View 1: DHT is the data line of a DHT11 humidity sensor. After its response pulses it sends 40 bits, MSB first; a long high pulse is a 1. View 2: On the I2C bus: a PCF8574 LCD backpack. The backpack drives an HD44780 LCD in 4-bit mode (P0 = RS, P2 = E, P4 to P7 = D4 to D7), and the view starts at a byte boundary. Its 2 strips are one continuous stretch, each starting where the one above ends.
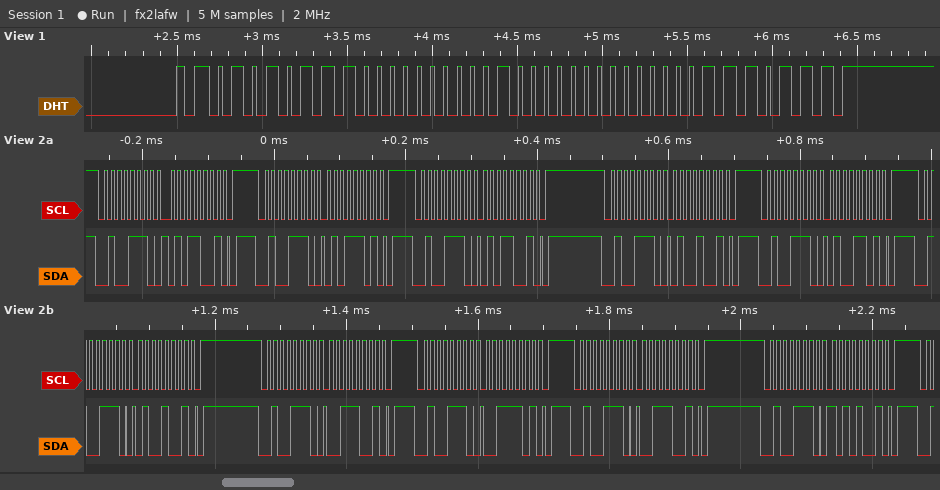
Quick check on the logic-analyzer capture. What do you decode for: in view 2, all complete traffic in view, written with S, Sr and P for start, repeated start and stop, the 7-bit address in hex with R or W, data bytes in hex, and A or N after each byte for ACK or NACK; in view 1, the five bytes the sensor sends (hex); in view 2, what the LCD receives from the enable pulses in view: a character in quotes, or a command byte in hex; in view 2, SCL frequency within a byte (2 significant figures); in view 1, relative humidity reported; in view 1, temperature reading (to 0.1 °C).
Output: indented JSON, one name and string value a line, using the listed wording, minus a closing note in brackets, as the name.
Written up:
{
  "in view 2, all complete traffic in view, written with S, Sr and P for start, repeated start and stop, the 7-bit address in hex with R or W, data bytes in hex, and A or N after each byte for ACK or NACK": "S 27W A 59 A P S 27W A 5D A P S 27W A 59 A P S 27W A 49 A P S 27W A 4D A P S 27W A 49 A P S 27W A 39 A P S 27W A 3D A P S 27W A 39 A P S 27W A A9 A P",
  "in view 1, the five bytes the sensor sends": "57 00 20 00 77",
  "in view 2, what the LCD receives from the enable pulses in view: a character in quotes, or a command byte in hex": "'T'",
  "in view 2, SCL frequency within a byte": "100 kHz",
  "in view 1, relative humidity reported": "87 %",
  "in view 1, temperature reading": "32.0 °C"
}
